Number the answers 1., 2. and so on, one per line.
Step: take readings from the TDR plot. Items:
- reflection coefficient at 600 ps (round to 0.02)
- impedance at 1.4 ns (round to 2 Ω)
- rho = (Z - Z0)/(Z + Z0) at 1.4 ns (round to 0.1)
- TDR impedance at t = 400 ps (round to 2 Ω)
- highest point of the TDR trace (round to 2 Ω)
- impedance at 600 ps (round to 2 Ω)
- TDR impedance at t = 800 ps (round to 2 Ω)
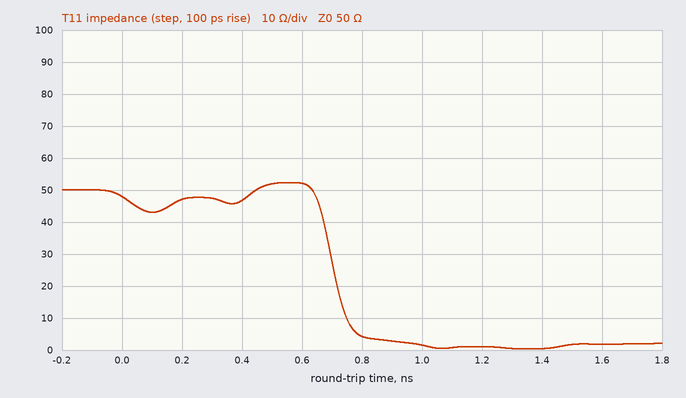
1. +0.02
2. 0 Ω
3. -1.0
4. 46 Ω
5. 52 Ω
6. 52 Ω
7. 4 Ω
